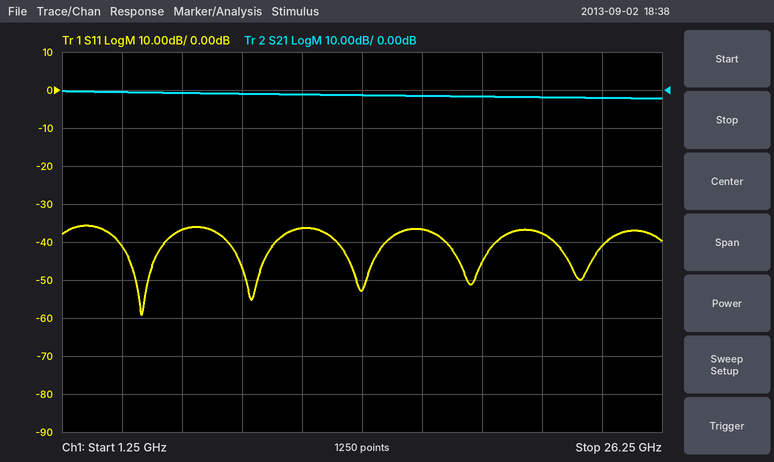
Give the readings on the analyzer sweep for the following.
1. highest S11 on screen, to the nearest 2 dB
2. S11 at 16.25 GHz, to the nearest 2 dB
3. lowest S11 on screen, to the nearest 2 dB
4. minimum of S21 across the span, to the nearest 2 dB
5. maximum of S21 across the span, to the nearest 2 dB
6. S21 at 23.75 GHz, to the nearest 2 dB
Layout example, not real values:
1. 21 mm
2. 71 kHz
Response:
1. -36 dB
2. -36 dB
3. -60 dB
4. -2 dB
5. 0 dB
6. -2 dB
